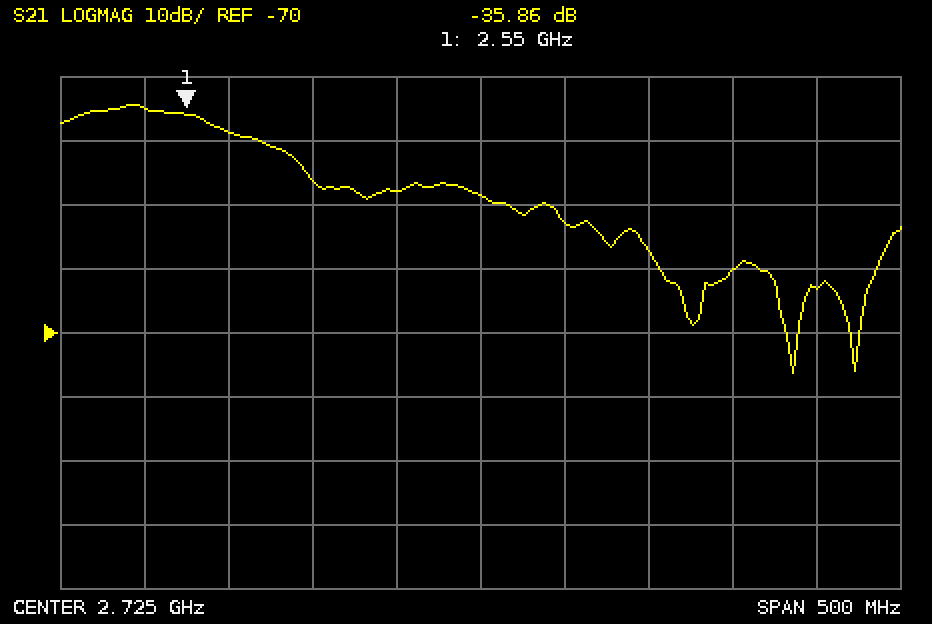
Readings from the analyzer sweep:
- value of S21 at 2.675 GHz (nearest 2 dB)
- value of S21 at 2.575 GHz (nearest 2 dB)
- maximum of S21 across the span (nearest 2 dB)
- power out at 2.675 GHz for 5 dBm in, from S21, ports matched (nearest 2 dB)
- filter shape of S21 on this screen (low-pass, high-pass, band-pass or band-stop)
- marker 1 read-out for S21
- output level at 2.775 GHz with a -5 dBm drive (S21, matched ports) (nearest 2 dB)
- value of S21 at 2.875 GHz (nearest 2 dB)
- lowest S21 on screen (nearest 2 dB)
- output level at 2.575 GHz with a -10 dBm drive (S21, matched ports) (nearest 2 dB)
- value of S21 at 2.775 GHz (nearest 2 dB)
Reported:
-48 dB
-38 dB
-34 dB
-42 dBm
low-pass
-35.86 dB
-58 dBm
-60 dB
-76 dB
-48 dBm
-52 dB
